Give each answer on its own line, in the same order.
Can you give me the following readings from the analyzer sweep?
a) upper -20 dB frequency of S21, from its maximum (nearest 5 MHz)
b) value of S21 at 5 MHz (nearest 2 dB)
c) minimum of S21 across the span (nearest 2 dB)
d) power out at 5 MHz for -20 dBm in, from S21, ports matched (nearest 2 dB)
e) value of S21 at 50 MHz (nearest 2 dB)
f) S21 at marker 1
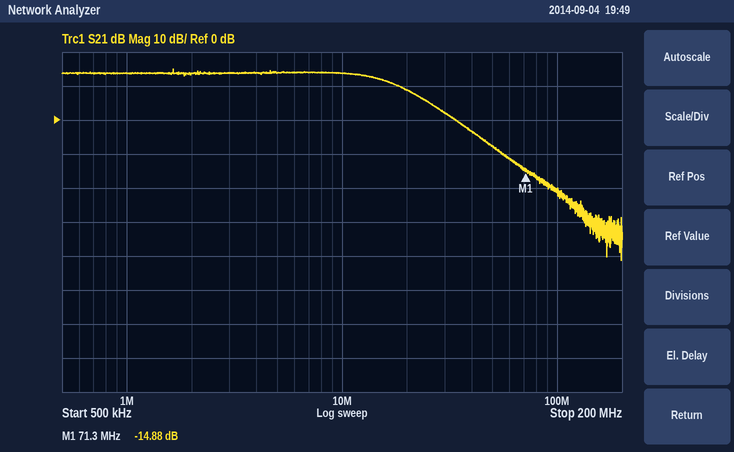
45 MHz
14 dB
-42 dB
-6 dBm
-8 dB
-14.88 dB
